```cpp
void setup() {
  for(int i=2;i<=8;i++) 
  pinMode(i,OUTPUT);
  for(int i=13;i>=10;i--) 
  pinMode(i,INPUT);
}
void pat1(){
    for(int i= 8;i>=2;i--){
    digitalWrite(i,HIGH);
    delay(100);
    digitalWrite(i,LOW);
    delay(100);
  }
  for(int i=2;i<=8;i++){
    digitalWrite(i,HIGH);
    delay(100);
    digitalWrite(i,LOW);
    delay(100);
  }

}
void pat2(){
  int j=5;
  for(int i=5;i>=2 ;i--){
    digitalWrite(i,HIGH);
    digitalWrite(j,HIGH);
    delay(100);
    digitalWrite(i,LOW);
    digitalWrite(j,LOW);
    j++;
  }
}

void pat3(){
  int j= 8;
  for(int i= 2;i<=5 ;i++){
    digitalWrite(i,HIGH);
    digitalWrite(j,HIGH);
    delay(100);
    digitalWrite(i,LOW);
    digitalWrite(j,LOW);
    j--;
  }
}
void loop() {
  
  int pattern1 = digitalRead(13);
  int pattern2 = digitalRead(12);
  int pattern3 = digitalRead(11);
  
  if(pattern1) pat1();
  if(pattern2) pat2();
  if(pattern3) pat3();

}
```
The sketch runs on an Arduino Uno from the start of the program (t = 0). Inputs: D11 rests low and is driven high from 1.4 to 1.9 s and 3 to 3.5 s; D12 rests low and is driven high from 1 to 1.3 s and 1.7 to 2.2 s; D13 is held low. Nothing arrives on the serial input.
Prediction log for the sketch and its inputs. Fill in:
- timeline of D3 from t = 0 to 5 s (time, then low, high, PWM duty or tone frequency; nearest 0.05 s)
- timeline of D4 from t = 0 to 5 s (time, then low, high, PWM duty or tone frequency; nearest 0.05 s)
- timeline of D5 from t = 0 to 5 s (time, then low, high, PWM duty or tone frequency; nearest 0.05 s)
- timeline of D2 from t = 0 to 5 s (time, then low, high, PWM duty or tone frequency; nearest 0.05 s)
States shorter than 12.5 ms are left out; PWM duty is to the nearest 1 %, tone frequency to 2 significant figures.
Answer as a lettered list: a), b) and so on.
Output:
a) 0 s low; 1.2 s high; 1.3 s low; 1.5 s high; 1.6 s low; 2 s high; 2.1 s low; 2.3 s high; 2.4 s low; 3.1 s high; 3.2 s low; 3.5 s high; 3.6 s low
b) 0 s low; 1.1 s high; 1.2 s low; 1.6 s high; 1.7 s low; 1.9 s high; 2 s low; 2.4 s high; 2.5 s low; 3.2 s high; 3.3 s low; 3.6 s high; 3.7 s low
c) 0 s low; 1 s high; 1.1 s low; 1.7 s high; 1.9 s low; 2.5 s high; 2.6 s low; 3.3 s high; 3.4 s low; 3.7 s high; 3.8 s low
d) 0 s low; 1.3 s high; 1.5 s low; 2.1 s high; 2.3 s low; 3 s high; 3.1 s low; 3.4 s high; 3.5 s low
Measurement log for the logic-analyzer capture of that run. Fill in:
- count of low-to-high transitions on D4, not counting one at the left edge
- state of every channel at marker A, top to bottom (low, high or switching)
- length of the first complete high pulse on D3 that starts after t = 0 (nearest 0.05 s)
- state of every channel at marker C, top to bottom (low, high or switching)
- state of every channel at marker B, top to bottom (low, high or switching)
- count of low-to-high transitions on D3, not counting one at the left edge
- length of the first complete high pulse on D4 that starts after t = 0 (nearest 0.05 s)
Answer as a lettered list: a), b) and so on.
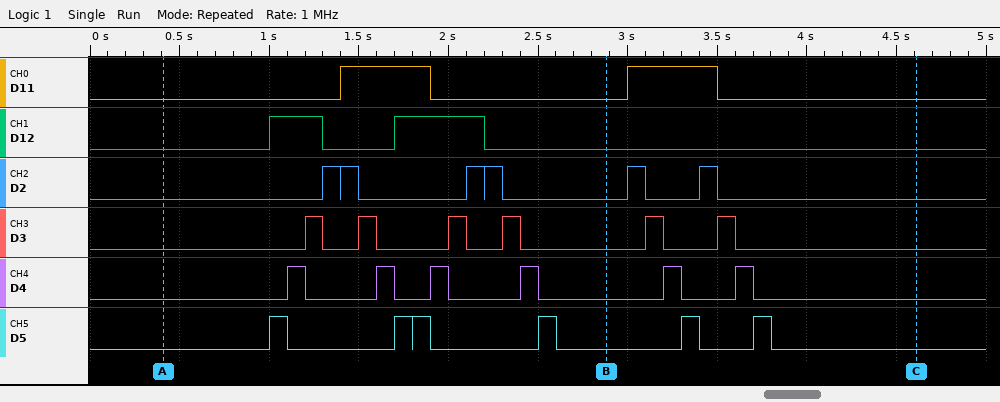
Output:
a) 6
b) D11 low, D12 low, D2 low, D3 low, D4 low, D5 low
c) 0.10 s
d) D11 low, D12 low, D2 low, D3 low, D4 low, D5 low
e) D11 low, D12 low, D2 low, D3 low, D4 low, D5 low
f) 6
g) 0.10 s
